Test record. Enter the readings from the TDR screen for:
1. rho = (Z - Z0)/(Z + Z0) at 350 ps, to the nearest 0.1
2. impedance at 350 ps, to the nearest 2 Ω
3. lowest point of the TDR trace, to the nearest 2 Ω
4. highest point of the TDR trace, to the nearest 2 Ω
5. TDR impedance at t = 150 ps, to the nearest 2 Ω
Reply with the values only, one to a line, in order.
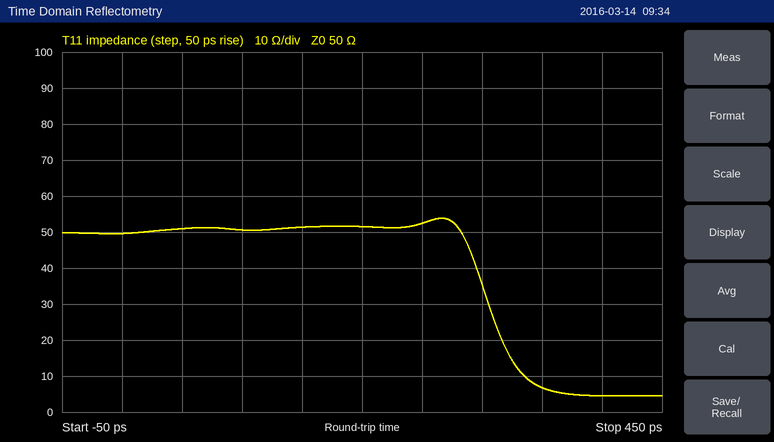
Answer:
-0.8
6 Ω
4 Ω
54 Ω
52 Ω
